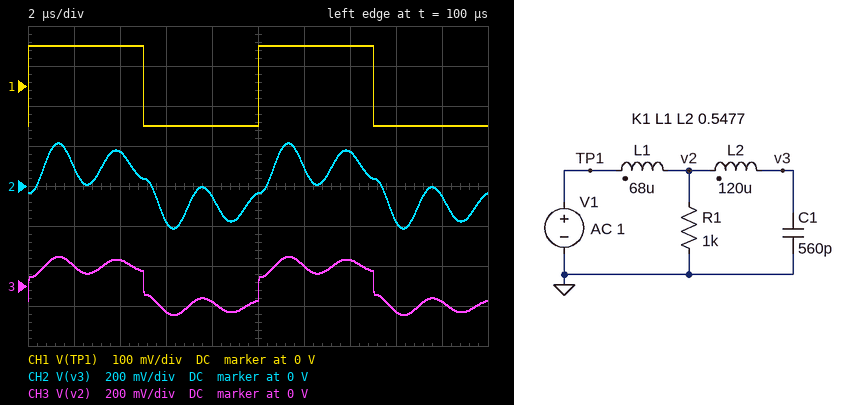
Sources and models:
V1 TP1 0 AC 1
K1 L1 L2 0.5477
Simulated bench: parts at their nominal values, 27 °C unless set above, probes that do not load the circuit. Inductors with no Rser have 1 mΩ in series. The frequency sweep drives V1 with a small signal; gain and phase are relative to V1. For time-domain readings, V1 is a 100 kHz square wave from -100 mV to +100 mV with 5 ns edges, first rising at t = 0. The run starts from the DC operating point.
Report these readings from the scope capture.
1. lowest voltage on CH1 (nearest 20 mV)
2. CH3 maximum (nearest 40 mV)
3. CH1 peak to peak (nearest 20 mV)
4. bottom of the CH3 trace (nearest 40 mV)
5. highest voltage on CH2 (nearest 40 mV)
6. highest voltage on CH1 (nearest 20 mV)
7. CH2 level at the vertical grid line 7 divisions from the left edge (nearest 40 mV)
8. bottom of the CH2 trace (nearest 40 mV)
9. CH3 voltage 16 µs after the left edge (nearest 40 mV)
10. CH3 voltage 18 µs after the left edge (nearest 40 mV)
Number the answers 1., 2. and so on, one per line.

1. -100 mV
2. 160 mV
3. 200 mV
4. -160 mV
5. 200 mV
6. 100 mV
7. 160 mV
8. -200 mV
9. -120 mV
10. -80 mV
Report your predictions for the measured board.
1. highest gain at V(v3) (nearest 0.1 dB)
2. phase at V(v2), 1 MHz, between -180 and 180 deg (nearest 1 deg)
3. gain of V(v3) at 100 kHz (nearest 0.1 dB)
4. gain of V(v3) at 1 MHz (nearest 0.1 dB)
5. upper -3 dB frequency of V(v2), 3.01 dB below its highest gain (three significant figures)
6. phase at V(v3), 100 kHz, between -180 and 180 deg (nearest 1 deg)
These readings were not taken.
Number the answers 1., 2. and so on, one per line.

1. 18.5 dB
2. -4 deg
3. 0.6 dB
4. -14.2 dB
5. 413 kHz
6. -4 deg
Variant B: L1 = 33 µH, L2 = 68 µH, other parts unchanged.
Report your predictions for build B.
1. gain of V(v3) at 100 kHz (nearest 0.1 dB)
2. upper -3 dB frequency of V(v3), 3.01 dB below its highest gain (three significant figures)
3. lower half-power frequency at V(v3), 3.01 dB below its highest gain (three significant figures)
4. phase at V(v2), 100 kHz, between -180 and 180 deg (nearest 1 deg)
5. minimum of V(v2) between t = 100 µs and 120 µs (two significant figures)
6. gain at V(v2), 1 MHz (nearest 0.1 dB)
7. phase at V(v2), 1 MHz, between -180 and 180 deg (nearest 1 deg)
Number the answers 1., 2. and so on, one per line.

1. 0.3 dB
2. 565 kHz
3. 522 kHz
4. -1 deg
5. -170 mV
6. -6.9 dB
7. 0 deg
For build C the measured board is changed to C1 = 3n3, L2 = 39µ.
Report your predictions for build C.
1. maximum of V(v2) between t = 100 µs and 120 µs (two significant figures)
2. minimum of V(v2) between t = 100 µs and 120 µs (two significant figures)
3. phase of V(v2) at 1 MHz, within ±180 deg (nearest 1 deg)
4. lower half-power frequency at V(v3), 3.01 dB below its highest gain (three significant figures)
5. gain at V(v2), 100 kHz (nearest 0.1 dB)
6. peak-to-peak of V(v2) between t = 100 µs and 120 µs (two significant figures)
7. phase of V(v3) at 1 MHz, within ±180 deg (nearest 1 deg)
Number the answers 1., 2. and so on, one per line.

1. 160 mV
2. -160 mV
3. -3 deg
4. 208 kHz
5. 1.3 dB
6. 320 mV
7. 167 deg
